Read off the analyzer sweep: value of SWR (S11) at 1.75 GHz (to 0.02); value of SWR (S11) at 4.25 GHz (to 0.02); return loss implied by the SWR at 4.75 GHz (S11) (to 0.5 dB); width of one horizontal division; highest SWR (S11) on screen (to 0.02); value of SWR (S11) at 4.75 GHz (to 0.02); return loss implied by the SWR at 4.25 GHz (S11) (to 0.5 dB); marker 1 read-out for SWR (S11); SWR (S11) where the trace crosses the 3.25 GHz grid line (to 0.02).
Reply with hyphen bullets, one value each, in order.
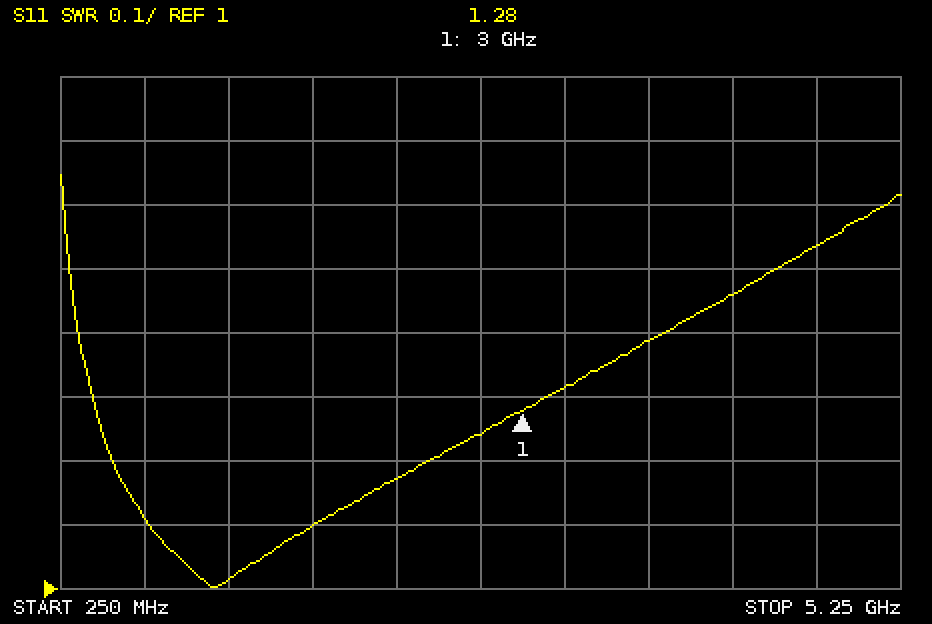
- 1.10
- 1.46
- 13.5 dB
- 500 MHz
- 1.64
- 1.54
- 14.5 dB
- 1.28
- 1.32
